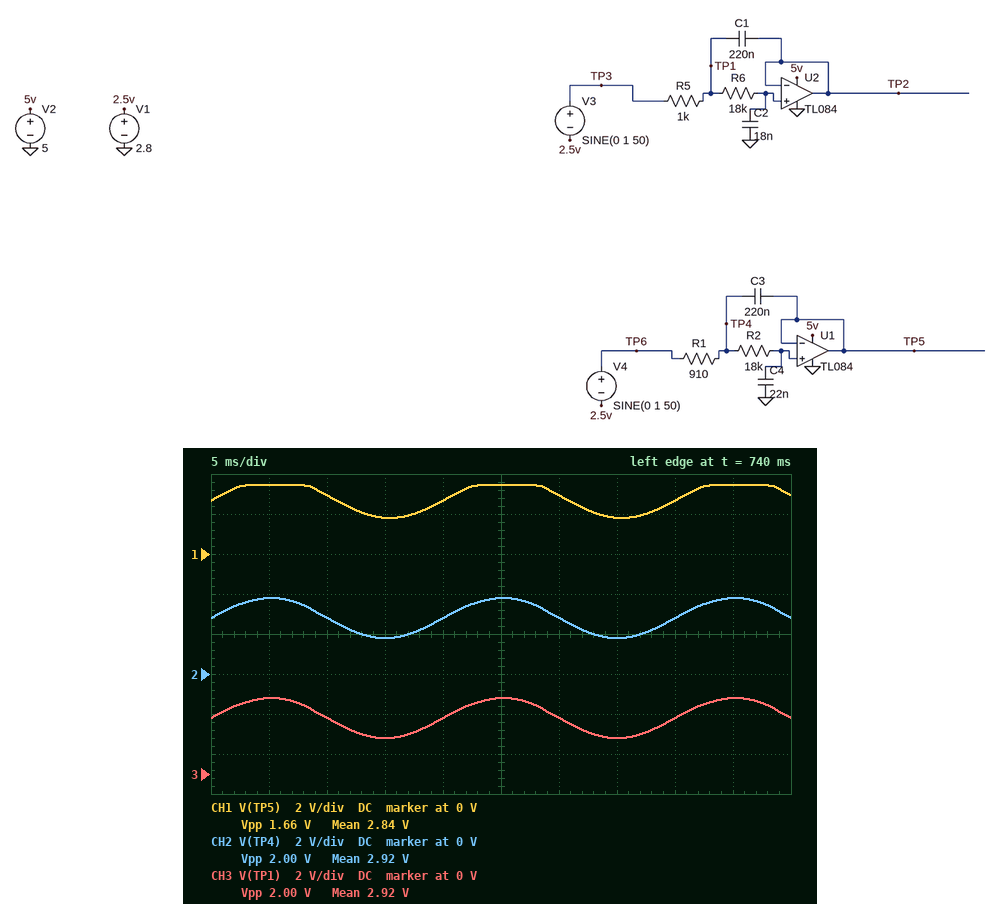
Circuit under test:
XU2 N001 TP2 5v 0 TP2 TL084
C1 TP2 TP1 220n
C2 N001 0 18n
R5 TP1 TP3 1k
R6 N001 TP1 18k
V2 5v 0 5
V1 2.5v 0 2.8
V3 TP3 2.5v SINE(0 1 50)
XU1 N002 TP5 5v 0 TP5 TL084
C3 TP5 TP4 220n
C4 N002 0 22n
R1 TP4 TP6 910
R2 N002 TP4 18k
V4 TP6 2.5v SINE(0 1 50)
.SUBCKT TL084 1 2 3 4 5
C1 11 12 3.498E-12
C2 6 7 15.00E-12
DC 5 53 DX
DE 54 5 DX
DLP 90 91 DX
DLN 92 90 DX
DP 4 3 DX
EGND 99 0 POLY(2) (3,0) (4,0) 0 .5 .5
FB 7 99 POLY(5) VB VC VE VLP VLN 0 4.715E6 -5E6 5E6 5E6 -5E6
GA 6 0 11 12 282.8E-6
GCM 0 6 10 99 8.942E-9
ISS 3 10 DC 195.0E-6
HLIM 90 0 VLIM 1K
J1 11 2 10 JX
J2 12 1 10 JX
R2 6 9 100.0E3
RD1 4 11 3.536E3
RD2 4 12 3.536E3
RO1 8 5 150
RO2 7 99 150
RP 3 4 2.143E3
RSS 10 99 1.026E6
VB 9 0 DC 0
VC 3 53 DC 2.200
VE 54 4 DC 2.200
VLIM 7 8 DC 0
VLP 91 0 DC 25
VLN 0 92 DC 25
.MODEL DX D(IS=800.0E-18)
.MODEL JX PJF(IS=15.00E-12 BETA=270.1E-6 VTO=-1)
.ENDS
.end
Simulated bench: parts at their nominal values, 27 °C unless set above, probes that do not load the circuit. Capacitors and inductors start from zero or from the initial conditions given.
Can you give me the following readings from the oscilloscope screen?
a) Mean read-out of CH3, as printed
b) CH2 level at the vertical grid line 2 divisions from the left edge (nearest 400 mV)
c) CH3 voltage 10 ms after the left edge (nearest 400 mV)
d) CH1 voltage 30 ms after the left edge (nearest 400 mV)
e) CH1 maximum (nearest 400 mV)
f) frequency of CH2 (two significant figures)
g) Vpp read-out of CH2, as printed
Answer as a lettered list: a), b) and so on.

a) 2.92 V
b) 2.8 V
c) 2.8 V
d) 2.8 V
e) 3.6 V
f) 50 Hz
g) 2.00 V
